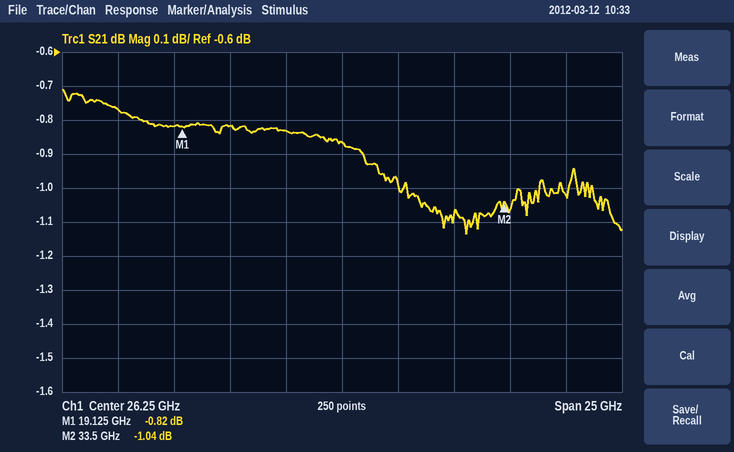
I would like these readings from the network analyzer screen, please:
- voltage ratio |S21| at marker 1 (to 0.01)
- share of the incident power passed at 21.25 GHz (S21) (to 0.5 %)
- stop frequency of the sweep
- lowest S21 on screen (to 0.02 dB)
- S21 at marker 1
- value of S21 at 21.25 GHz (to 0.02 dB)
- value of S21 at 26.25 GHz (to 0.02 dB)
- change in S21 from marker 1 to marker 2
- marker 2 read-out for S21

0.91
83.0 %
38.75 GHz
-1.14 dB
-0.82 dB
-0.82 dB
-0.86 dB
-0.22 dB
-1.04 dB
